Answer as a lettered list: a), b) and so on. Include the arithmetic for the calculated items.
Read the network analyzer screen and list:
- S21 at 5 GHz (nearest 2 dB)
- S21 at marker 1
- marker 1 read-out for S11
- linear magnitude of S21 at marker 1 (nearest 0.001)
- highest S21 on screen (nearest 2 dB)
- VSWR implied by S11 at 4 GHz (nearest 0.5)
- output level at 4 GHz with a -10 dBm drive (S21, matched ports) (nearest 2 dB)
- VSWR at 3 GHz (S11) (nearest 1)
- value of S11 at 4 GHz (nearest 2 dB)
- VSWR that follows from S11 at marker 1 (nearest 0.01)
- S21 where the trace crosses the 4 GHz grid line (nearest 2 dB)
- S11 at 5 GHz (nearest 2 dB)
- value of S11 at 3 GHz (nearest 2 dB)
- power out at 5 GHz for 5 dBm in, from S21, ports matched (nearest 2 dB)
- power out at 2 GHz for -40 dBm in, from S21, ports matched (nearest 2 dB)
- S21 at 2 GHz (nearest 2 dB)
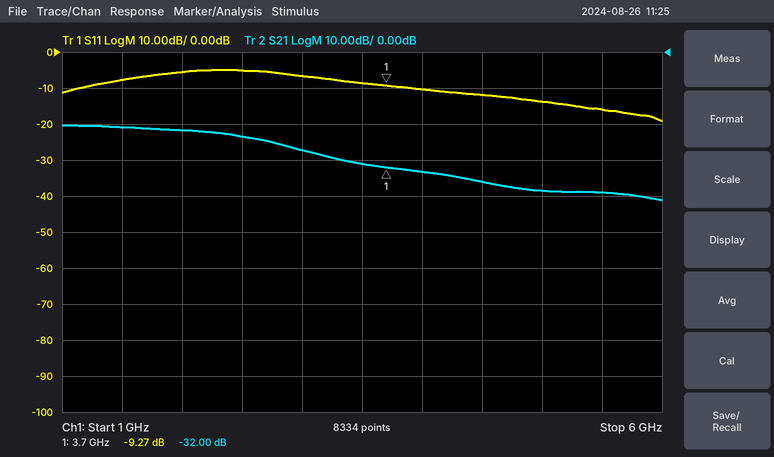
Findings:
a) -38 dB
b) -32.00 dB
c) -9.27 dB
d) 10^(-32/20) ≈ 0.025
e) -20 dB
f) |Γ| = 10^(-10/20) = 0.3162; VSWR = (1 + 0.3162)/(1 − 0.3162) ≈ 1.92, so 2.0 to the nearest 0.5
g) -10 dBm + (-34 dB) = -44 dBm
h) |Γ| = 10^(-6/20) = 0.5012; VSWR = (1 + 0.5012)/(1 − 0.5012) ≈ 3
i) -10 dB
j) (1 + 0.3440)/(1 − 0.3440) ≈ 2.05
k) -34 dB
l) -14 dB
m) -6 dB
n) 5 dBm + (-38 dB) = -34 dBm
o) -40 dBm + (-22 dB) = -62 dBm
p) -22 dB
